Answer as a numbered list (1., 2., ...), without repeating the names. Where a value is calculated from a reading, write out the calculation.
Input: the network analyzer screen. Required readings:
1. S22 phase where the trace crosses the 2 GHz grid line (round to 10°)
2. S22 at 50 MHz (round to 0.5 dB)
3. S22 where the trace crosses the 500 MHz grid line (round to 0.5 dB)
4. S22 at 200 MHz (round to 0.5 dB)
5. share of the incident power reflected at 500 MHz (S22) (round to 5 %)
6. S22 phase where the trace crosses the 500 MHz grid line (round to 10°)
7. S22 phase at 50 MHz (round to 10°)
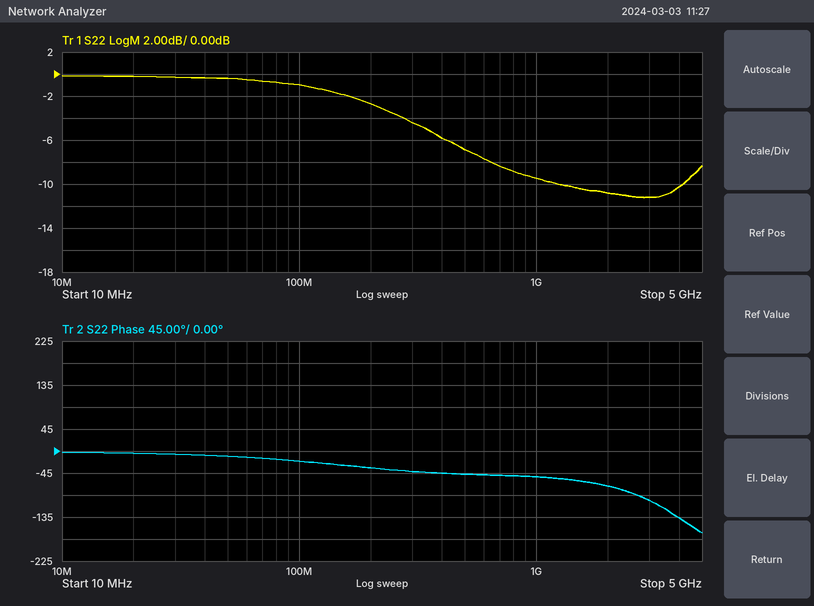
1. -70°
2. -0.5 dB
3. -7.0 dB
4. -2.5 dB
5. 10^(-7/10) ≈ 20 %
6. -50°
7. -10°
